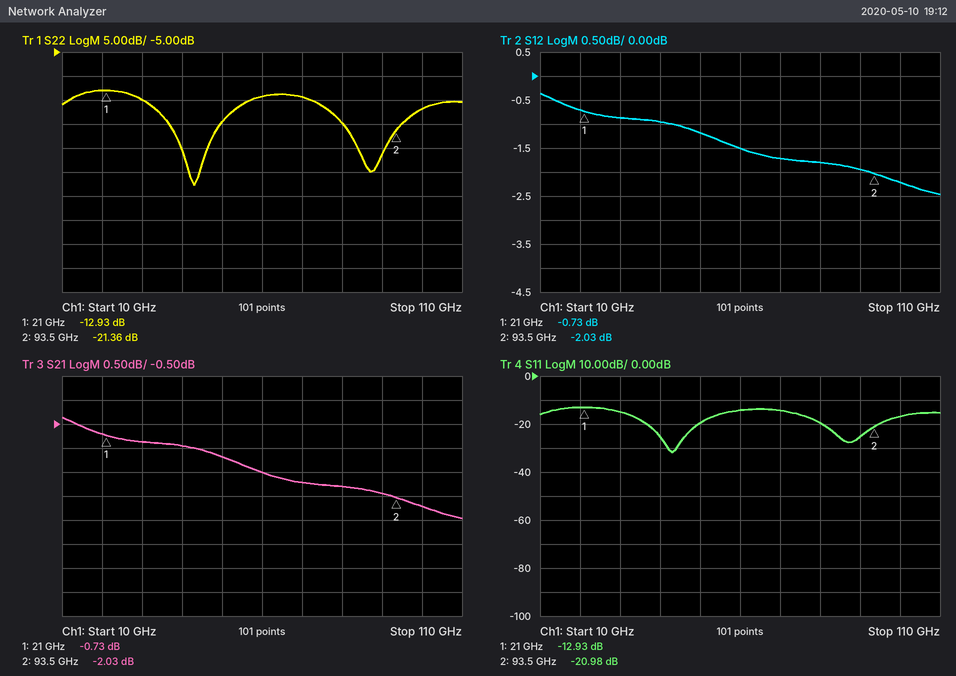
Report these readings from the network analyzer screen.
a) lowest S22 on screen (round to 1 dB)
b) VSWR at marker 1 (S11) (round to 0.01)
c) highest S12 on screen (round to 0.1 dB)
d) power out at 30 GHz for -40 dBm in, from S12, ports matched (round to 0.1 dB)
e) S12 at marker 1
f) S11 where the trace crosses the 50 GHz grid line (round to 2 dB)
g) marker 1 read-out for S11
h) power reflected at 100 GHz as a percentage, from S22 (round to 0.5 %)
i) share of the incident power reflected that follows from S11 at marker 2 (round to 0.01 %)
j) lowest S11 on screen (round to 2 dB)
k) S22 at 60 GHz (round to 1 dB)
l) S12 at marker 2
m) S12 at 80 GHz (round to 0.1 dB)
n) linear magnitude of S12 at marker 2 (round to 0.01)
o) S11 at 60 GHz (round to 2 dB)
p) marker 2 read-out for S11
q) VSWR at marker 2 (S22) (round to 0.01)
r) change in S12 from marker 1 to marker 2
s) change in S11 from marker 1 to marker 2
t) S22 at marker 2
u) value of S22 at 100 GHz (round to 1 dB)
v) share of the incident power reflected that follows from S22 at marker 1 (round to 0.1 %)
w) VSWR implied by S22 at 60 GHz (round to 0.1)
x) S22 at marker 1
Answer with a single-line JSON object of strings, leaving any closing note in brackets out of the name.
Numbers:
{"lowest S22 on screen": "-33 dB", "VSWR at marker 1 (S11)": "1.58", "highest S12 on screen": "-0.4 dB", "power out at 30 GHz for -40 dBm in, from S12, ports matched": "-40.9 dBm", "S12 at marker 1": "-0.73 dB", "S11 where the trace crosses the 50 GHz grid line": "-20 dB", "marker 1 read-out for S11": "-12.93 dB", "power reflected at 100 GHz as a percentage, from S22": "2.0 %", "share of the incident power reflected that follows from S11 at marker 2": "0.80 %", "lowest S11 on screen": "-32 dB", "S22 at 60 GHz": "-14 dB", "S12 at marker 2": "-2.03 dB", "S12 at 80 GHz": "-1.8 dB", "linear magnitude of S12 at marker 2": "0.79", "S11 at 60 GHz": "-14 dB", "marker 2 read-out for S11": "-20.98 dB", "VSWR at marker 2 (S22)": "1.19", "change in S12 from marker 1 to marker 2": "-1.30 dB", "change in S11 from marker 1 to marker 2": "-8.05 dB", "S22 at marker 2": "-21.36 dB", "value of S22 at 100 GHz": "-17 dB", "share of the incident power reflected that follows from S22 at marker 1": "5.1 %", "VSWR implied by S22 at 60 GHz": "1.5", "S22 at marker 1": "-12.93 dB"}
